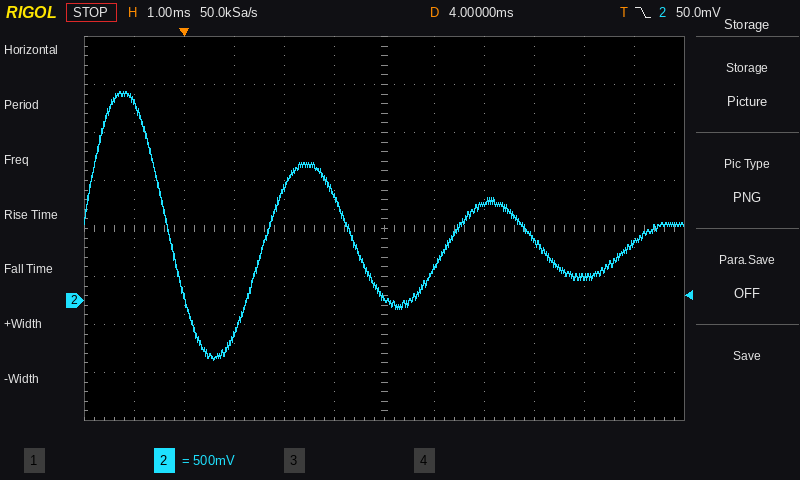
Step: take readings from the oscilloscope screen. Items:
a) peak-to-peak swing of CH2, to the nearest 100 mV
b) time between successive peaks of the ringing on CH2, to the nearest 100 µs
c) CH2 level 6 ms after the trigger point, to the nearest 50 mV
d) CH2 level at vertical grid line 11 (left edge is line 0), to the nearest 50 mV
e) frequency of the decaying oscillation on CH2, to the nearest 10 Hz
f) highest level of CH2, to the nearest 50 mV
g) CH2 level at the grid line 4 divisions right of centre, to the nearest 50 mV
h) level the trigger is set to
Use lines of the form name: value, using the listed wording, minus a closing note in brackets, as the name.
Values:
peak-to-peak swing of CH2, to the nearest 100 mV: 2.80 V
time between successive peaks of the ringing on CH2, to the nearest 100 µs: 3.7 ms
CH2 level 6 ms after the trigger point, to the nearest 50 mV: 1.00 V
CH2 level at vertical grid line 11 (left edge is line 0), to the nearest 50 mV: 600 mV
frequency of the decaying oscillation on CH2, to the nearest 10 Hz: 270 Hz
highest level of CH2, to the nearest 50 mV: 2.20 V
CH2 level at the grid line 4 divisions right of centre, to the nearest 50 mV: 250 mV
level the trigger is set to: 50.0 mV
